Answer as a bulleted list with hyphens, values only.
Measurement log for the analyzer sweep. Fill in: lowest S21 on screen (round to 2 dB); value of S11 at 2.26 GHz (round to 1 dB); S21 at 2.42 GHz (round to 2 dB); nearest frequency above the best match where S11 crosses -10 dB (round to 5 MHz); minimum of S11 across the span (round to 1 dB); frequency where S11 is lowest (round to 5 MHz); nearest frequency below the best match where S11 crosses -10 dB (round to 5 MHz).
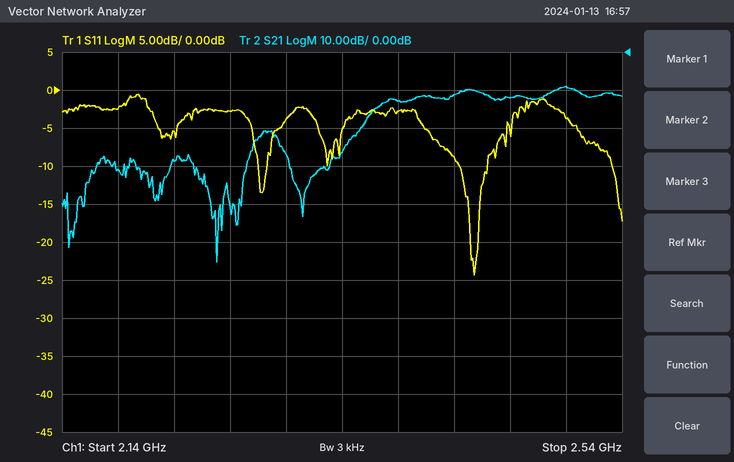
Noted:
- -56 dB
- -3 dB
- -12 dB
- 2.445 GHz
- -24 dB
- 2.435 GHz
- 2.425 GHz
